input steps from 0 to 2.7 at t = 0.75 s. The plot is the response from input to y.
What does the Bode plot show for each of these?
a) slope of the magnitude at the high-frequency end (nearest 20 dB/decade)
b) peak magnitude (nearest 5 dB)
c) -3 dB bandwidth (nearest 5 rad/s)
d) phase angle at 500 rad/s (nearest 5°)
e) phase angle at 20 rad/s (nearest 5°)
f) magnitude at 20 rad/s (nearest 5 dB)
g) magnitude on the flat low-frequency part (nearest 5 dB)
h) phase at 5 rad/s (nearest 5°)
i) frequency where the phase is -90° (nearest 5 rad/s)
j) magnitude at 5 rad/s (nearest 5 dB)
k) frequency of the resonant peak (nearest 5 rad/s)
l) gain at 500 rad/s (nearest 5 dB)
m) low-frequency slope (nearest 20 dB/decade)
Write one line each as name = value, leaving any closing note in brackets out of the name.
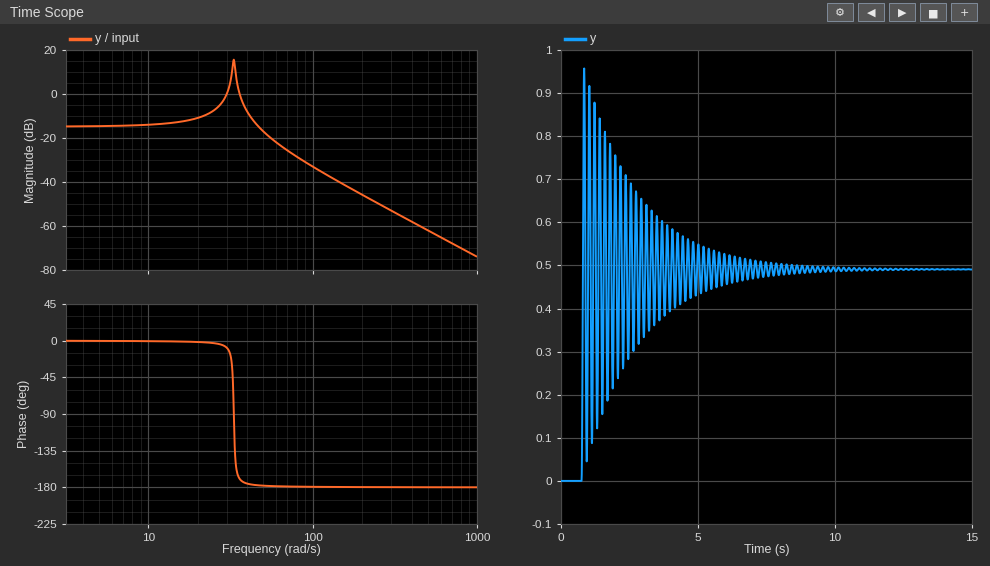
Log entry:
slope of the magnitude at the high-frequency end = -40 dB/decade
peak magnitude = 15 dB
-3 dB bandwidth = 50 rad/s
phase angle at 500 rad/s = -180°
phase angle at 20 rad/s = 0°
magnitude at 20 rad/s = -10 dB
magnitude on the flat low-frequency part = -15 dB
phase at 5 rad/s = 0°
frequency where the phase is -90° = 35 rad/s
magnitude at 5 rad/s = -15 dB
frequency of the resonant peak = 35 rad/s
gain at 500 rad/s = -60 dB
low-frequency slope = 0 dB/decade
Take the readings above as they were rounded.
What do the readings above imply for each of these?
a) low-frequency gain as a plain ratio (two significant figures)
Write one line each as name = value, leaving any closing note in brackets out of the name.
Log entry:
low-frequency gain as a plain ratio = 0.18
